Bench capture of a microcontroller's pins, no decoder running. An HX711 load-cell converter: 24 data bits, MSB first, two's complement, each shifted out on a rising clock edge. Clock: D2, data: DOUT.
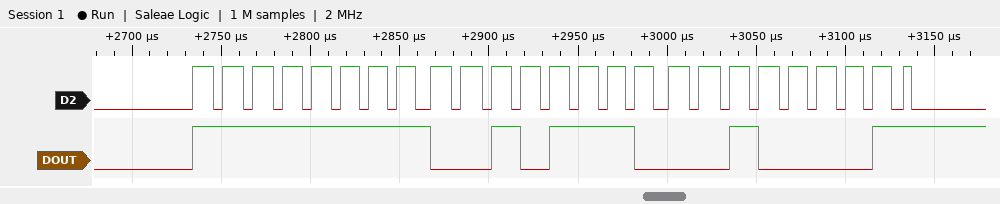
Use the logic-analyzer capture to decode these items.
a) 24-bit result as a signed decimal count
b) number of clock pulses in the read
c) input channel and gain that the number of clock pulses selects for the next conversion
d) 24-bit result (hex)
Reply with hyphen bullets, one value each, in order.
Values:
- -53727
- 25
- channel A, gain 128
- 0xFF2E21
